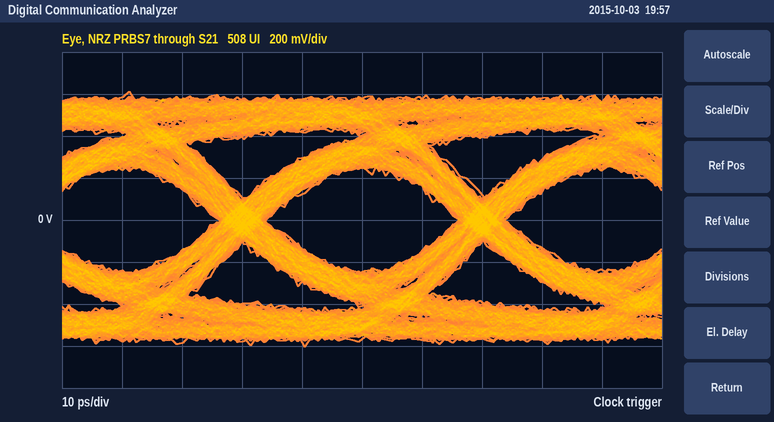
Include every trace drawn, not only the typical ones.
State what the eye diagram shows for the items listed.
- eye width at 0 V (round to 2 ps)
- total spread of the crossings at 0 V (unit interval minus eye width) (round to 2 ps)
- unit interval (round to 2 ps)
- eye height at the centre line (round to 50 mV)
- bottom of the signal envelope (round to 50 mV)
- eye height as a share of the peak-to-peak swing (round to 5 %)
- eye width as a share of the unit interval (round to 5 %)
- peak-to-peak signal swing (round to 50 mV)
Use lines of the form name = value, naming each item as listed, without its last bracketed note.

eye width at 0 V = 32 ps
total spread of the crossings at 0 V (unit interval minus eye width) = 8 ps
unit interval = 40 ps
eye height at the centre line = 500 mV
bottom of the signal envelope = -600 mV
eye height as a share of the peak-to-peak swing = 40 %
eye width as a share of the unit interval = 80 %
peak-to-peak signal swing = 1.20 V
